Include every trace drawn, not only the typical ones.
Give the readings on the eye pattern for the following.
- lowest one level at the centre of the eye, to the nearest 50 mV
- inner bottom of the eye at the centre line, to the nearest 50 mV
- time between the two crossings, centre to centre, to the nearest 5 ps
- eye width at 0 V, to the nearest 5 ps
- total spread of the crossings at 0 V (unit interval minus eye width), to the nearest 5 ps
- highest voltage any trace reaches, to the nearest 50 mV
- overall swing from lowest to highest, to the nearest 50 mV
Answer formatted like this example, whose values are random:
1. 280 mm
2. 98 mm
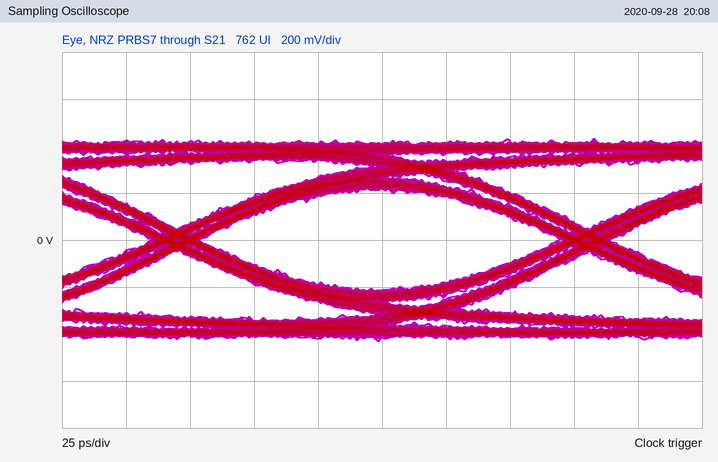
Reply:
1. 200 mV
2. -200 mV
3. 160 ps
4. 140 ps
5. 20 ps
6. 450 mV
7. 850 mV
